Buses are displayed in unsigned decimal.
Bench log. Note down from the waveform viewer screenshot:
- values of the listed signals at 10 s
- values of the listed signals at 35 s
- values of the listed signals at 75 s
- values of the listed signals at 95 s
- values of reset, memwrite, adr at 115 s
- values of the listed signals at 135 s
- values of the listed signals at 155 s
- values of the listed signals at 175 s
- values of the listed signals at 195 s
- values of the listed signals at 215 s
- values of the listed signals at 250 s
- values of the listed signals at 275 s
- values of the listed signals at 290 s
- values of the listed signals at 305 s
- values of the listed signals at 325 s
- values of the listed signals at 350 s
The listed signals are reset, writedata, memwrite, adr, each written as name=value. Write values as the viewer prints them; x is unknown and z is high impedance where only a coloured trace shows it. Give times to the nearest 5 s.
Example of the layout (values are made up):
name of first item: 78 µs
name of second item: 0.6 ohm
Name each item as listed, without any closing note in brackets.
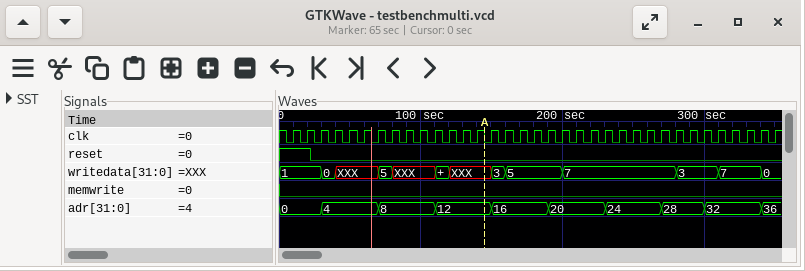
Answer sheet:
values of the listed signals at 10 s: reset=1, writedata=1, memwrite=0, adr=0
values of the listed signals at 35 s: reset=0, writedata=0, memwrite=0, adr=4
values of the listed signals at 75 s: reset=0, writedata=5, memwrite=0, adr=8
values of the listed signals at 95 s: reset=0, writedata=XXX, memwrite=0, adr=8
values of reset, memwrite, adr at 115 s: reset=0, memwrite=0, adr=12
values of the listed signals at 135 s: reset=0, writedata=XXX, memwrite=0, adr=12
values of the listed signals at 155 s: reset=0, writedata=3, memwrite=0, adr=16
values of the listed signals at 175 s: reset=0, writedata=5, memwrite=0, adr=16
values of the listed signals at 195 s: reset=0, writedata=5, memwrite=0, adr=20
values of the listed signals at 215 s: reset=0, writedata=7, memwrite=0, adr=20
values of the listed signals at 250 s: reset=0, writedata=7, memwrite=0, adr=24
values of the listed signals at 275 s: reset=0, writedata=7, memwrite=0, adr=28
values of the listed signals at 290 s: reset=0, writedata=3, memwrite=0, adr=28
values of the listed signals at 305 s: reset=0, writedata=3, memwrite=0, adr=32
values of the listed signals at 325 s: reset=0, writedata=7, memwrite=0, adr=32
values of the listed signals at 350 s: reset=0, writedata=0, memwrite=0, adr=36
